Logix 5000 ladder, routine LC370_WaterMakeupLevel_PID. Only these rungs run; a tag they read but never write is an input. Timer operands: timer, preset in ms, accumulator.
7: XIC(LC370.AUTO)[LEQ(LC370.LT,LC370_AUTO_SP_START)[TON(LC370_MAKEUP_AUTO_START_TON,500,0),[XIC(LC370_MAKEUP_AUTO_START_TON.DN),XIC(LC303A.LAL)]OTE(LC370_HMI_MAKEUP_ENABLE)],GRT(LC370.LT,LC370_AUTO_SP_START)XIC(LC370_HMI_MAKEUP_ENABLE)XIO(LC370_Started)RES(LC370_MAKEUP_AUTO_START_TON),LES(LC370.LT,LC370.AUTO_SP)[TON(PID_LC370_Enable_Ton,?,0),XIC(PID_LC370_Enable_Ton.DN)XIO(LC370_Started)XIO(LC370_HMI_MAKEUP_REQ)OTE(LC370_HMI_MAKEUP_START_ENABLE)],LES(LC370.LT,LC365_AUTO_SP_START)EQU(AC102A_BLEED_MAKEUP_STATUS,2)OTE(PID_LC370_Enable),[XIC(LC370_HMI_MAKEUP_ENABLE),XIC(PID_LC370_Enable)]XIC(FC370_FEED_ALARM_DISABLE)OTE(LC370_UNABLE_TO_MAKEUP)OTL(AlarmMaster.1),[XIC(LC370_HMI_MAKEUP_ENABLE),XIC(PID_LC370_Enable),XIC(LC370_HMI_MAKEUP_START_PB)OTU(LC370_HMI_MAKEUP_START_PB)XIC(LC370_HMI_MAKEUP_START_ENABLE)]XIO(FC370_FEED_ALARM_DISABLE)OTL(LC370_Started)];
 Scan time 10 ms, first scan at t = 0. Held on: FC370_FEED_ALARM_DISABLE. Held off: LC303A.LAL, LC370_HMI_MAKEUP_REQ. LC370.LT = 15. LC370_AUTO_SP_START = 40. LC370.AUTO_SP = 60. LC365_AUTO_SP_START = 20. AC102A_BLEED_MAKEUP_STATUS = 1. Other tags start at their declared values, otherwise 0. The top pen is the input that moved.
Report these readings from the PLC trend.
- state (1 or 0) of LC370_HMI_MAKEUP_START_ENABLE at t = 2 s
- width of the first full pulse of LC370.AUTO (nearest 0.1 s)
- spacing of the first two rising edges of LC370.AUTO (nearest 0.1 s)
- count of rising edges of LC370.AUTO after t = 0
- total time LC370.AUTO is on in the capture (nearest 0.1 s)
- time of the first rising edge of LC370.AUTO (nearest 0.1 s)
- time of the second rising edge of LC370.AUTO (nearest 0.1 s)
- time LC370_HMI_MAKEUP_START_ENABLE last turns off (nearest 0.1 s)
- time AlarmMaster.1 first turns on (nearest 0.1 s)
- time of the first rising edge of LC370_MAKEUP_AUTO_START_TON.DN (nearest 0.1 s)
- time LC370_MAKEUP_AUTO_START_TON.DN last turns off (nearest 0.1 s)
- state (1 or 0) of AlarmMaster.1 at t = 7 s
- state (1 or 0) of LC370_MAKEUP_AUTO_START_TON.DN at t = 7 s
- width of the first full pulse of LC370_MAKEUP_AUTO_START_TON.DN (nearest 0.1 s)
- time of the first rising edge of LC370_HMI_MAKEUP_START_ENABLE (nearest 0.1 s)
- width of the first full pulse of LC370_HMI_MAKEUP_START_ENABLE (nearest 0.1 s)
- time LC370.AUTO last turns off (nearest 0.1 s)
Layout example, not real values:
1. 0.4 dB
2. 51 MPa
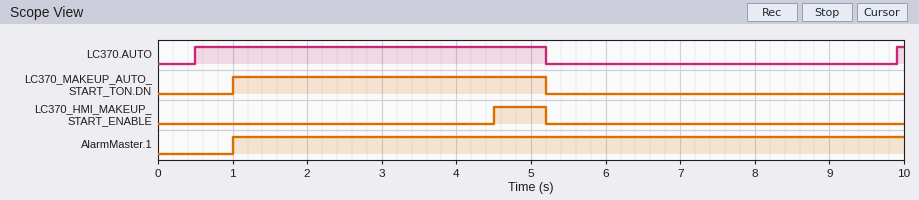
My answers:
1. 0
2. 4.7 s
3. 9.4 s
4. 2
5. 4.8 s
6. 0.5 s
7. 9.9 s
8. 5.2 s
9. 1.0 s
10. 1.0 s
11. 5.2 s
12. 1
13. 0
14. 4.2 s
15. 4.5 s
16. 0.7 s
17. 5.2 s
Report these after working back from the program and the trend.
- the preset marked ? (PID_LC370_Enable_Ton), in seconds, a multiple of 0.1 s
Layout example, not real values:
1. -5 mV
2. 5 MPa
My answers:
1. 4.0 s
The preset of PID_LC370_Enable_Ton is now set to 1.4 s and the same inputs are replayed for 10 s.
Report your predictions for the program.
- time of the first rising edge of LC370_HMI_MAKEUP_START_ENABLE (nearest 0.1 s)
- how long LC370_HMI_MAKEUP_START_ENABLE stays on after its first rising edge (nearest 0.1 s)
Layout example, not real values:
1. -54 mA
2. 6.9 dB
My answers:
1. 1.9 s
2. 3.3 s
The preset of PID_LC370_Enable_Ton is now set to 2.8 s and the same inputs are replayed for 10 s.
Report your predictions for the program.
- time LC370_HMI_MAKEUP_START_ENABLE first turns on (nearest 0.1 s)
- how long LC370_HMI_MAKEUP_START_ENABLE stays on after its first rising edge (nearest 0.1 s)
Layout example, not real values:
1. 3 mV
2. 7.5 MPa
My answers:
1. 3.3 s
2. 1.9 s
